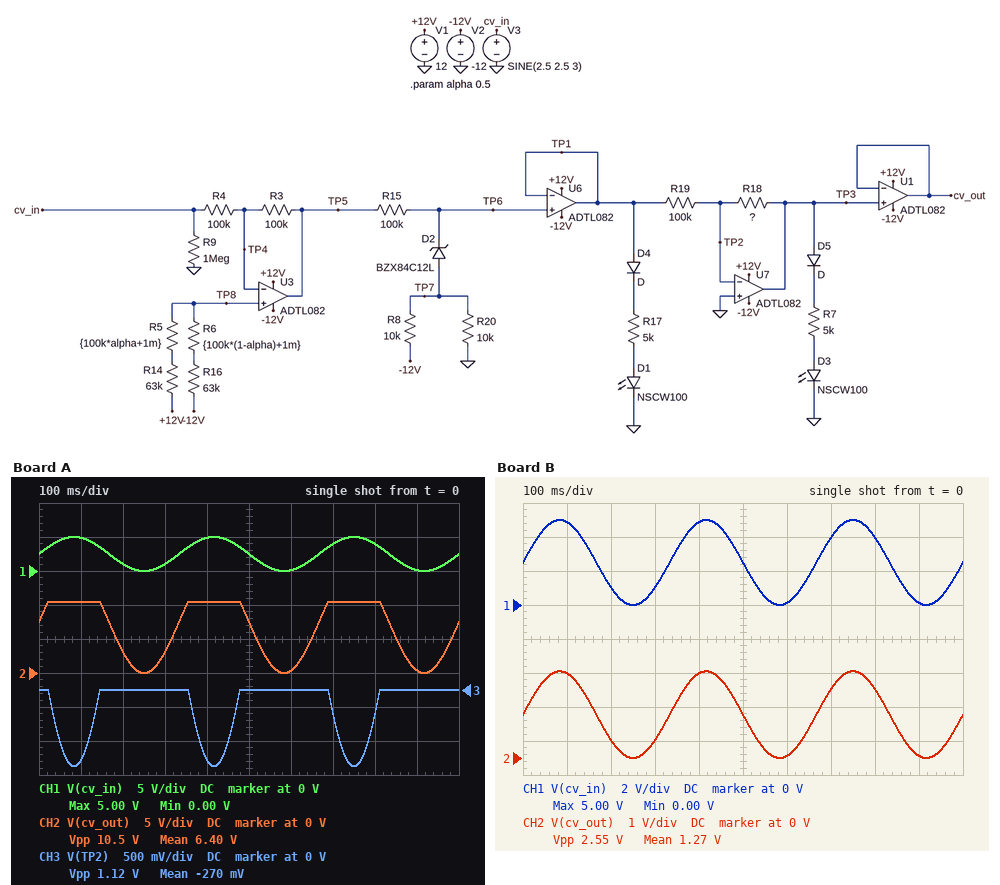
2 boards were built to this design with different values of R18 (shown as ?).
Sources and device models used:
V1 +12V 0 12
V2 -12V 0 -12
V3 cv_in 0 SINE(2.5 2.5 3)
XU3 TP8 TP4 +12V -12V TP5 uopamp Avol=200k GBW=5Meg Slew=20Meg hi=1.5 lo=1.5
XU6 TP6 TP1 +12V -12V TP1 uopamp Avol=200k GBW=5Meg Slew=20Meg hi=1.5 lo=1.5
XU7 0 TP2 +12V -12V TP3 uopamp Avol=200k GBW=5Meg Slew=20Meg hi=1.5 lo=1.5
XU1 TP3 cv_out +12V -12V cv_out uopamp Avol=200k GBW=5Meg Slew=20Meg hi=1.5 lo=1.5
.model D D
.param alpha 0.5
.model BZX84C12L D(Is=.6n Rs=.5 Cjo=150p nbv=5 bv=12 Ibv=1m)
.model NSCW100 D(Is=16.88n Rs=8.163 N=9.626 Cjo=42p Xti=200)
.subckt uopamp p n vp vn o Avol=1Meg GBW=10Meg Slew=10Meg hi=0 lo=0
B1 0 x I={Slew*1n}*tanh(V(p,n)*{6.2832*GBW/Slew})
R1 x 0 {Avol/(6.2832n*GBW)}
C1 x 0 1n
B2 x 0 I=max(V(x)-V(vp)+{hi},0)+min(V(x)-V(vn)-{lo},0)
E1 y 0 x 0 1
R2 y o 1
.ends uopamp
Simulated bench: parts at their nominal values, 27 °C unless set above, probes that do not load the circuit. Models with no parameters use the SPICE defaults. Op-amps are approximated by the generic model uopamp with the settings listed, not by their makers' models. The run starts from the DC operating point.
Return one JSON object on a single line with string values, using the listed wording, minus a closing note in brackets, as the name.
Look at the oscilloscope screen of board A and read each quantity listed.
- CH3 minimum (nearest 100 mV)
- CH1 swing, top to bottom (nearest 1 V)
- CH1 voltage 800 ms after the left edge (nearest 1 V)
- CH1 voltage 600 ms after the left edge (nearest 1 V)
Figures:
{"CH3 minimum": "-1.1 V", "CH1 swing, top to bottom": "5 V", "CH1 voltage 800 ms after the left edge": "4 V", "CH1 voltage 600 ms after the left edge": "0 V"}
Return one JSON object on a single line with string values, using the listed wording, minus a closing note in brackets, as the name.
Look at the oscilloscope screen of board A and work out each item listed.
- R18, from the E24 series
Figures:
{"R18, from the E24 series": "300 kΩ"}
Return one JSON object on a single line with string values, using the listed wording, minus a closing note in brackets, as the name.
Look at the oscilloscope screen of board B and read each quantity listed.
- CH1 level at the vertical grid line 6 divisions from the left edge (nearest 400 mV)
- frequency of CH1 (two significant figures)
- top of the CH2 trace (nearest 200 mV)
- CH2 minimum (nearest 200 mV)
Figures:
{"CH1 level at the vertical grid line 6 divisions from the left edge": "0 V", "frequency of CH1": "3.0 Hz", "top of the CH2 trace": "2.6 V", "CH2 minimum": "0 V"}
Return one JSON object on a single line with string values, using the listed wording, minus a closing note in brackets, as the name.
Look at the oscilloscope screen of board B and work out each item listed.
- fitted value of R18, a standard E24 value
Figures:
{"fitted value of R18, a standard E24 value": "51 kΩ"}
